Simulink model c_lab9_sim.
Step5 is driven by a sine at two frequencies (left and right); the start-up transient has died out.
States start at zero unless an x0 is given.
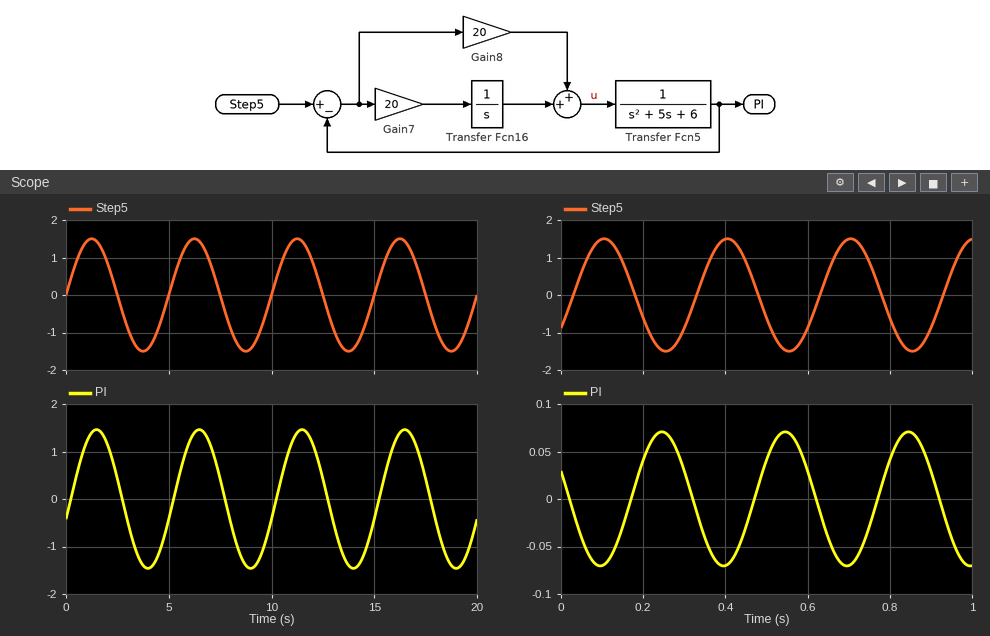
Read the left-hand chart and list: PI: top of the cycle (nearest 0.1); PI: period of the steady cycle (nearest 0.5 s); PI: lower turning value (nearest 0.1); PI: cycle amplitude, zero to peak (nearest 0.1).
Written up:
1.5
5.0 s
-1.5
1.5
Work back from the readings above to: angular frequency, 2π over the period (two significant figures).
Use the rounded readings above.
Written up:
1.3 rad/s
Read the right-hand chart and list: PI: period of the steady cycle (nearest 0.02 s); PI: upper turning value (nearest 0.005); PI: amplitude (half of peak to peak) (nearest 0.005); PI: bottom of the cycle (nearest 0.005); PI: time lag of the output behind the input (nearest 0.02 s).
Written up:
0.30 s
0.070
0.070
-0.070
0.14 s
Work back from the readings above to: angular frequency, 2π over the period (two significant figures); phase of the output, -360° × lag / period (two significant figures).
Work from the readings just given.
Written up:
21 rad/s
-170°
